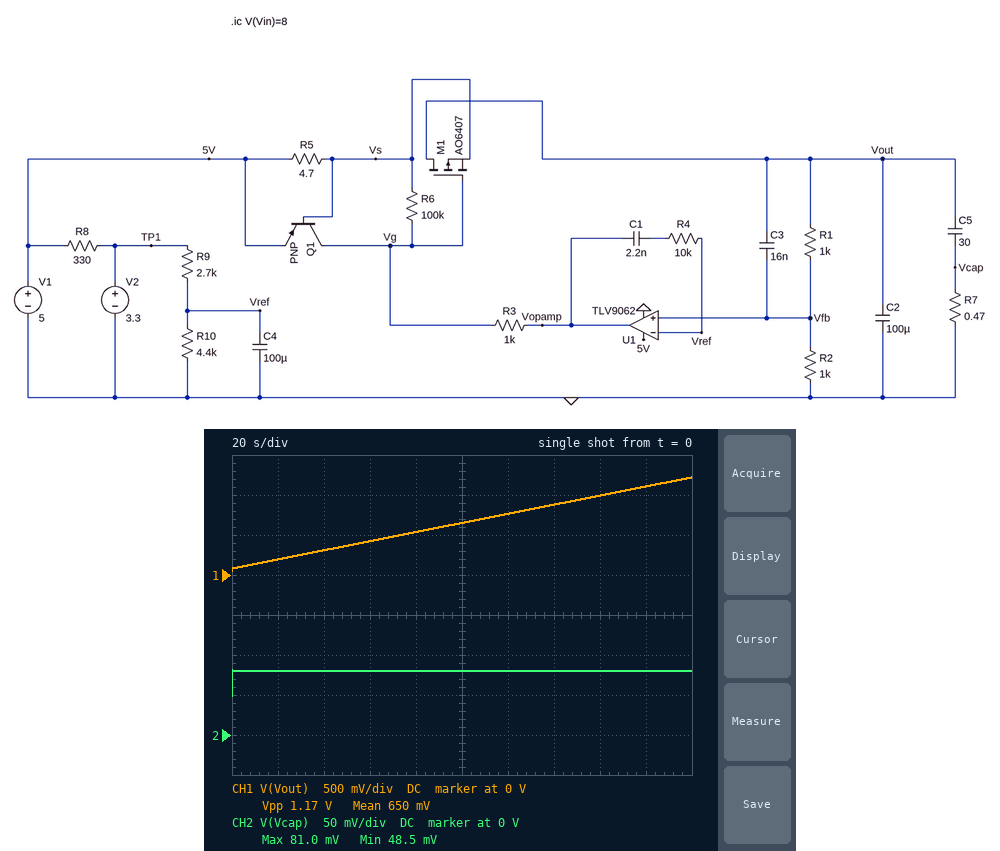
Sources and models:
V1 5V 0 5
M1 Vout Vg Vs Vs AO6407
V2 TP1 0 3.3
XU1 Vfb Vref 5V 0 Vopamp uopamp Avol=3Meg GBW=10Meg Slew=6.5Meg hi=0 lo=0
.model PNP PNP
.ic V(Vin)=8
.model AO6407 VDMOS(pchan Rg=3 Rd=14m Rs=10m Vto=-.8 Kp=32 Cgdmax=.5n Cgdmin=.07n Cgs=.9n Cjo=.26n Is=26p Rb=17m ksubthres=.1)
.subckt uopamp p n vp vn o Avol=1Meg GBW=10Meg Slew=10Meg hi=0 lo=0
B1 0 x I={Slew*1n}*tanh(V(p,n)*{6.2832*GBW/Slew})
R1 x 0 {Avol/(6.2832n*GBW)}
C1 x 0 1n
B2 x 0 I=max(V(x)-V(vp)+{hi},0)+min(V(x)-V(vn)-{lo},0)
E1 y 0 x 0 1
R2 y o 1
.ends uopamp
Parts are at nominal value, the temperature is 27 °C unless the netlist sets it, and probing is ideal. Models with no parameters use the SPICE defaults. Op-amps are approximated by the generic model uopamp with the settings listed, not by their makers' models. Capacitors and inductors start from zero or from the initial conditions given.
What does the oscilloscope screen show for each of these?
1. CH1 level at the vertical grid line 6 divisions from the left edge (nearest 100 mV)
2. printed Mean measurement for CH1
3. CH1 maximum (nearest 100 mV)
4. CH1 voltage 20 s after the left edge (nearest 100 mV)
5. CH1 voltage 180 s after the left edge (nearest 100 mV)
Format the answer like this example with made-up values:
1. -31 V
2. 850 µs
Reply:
1. 800 mV
2. 650 mV
3. 1.2 V
4. 200 mV
5. 1.1 V
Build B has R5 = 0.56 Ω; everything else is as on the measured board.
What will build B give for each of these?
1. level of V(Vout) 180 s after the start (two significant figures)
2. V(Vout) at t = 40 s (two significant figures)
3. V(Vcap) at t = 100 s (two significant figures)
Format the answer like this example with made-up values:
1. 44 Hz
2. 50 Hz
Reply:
1. 4.1 V
2. 2.6 V
3. 89 mV
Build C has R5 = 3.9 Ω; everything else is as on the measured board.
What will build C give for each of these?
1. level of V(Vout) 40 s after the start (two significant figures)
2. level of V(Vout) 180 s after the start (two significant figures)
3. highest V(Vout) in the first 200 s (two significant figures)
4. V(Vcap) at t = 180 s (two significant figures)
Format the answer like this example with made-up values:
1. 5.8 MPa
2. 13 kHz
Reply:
1. 370 mV
2. 1.3 V
3. 1.5 V
4. 97 mV
